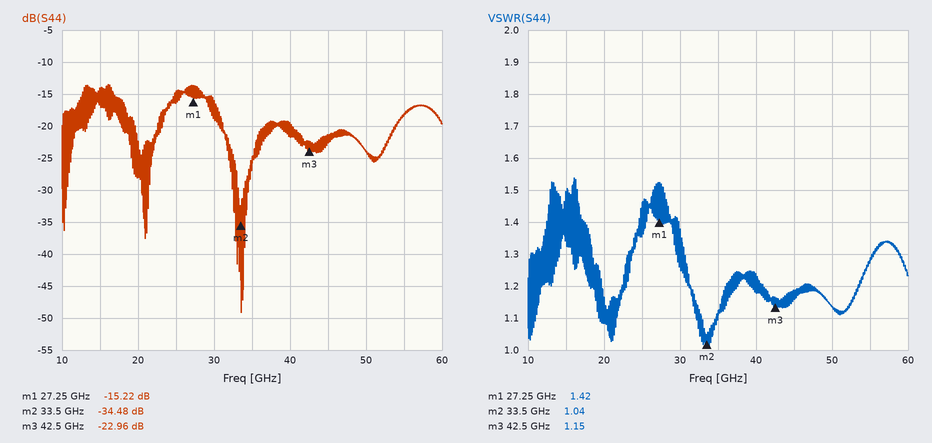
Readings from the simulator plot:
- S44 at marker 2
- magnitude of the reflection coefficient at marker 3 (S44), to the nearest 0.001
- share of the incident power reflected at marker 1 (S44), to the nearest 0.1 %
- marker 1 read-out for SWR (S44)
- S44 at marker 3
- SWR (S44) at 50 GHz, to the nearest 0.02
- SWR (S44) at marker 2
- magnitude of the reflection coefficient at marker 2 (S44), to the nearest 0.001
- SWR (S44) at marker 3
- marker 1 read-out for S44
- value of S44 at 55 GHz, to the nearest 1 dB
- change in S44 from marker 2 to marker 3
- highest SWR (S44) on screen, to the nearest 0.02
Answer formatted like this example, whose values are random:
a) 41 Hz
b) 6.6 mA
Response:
a) -34.48 dB
b) 0.071
c) 3.0 %
d) 1.42
e) -22.96 dB
f) 1.14
g) 1.04
h) 0.019
i) 1.15
j) -15.22 dB
k) -18 dB
l) 11.52 dB
m) 1.54
